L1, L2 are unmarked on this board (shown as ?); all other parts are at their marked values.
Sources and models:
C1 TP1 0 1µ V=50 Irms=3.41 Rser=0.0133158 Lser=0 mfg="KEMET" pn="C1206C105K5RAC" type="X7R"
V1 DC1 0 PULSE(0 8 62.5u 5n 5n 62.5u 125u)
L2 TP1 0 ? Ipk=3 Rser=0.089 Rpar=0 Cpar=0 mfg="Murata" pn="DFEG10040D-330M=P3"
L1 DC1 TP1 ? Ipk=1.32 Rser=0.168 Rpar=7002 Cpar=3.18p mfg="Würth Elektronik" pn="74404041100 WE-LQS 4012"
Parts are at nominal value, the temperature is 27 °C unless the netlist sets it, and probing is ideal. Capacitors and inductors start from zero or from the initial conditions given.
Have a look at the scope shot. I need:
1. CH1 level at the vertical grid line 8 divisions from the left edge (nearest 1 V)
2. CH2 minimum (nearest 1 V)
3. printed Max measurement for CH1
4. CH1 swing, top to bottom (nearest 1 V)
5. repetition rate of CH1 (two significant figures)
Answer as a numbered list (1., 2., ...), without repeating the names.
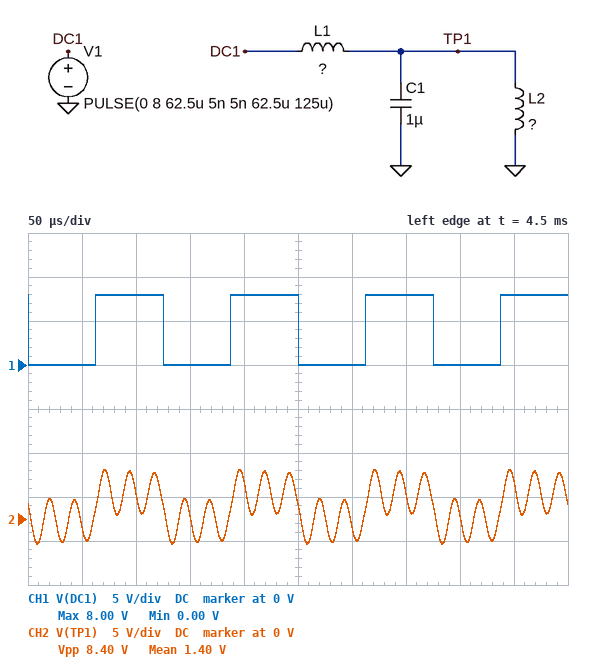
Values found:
1. 0 V
2. -3 V
3. 8.00 V
4. 8 V
5. 8.0 kHz
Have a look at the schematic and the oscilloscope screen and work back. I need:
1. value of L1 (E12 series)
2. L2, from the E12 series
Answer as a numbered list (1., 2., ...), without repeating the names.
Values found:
1. 33 µH
2. 22 µH
